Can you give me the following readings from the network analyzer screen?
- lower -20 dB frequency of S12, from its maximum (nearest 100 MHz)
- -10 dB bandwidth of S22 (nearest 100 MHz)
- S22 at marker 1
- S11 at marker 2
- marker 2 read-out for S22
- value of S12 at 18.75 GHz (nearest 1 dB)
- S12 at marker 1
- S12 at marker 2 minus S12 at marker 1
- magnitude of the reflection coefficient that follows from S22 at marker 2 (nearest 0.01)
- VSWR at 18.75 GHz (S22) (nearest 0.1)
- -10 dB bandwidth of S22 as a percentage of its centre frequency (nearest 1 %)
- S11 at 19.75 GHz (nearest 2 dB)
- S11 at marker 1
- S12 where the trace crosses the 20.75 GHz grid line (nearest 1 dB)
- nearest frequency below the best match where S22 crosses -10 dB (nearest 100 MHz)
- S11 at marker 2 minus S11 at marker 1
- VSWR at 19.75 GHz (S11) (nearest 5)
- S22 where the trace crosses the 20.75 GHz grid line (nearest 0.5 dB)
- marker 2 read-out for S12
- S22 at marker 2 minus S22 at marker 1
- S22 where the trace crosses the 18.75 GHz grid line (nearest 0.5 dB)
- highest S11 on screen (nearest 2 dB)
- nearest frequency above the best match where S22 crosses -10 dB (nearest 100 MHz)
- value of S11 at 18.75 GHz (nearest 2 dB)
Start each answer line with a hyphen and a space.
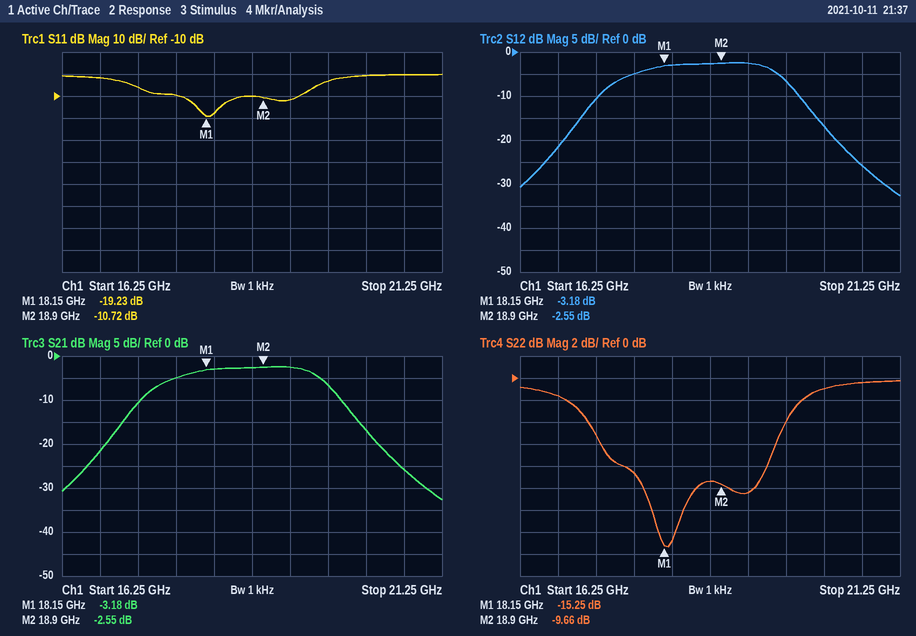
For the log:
- 16.7 GHz
- 700 MHz
- -15.25 dB
- -10.72 dB
- -9.66 dB
- -3 dB
- -3.18 dB
- 0.63 dB
- 0.33
- 2.0
- 4 %
- -4 dB
- -19.23 dB
- -26 dB
- 17.9 GHz
- 8.51 dB
- 5
- -0.5 dB
- -2.55 dB
- 5.59 dB
- -9.5 dB
- 0 dB
- 18.6 GHz
- -10 dB
